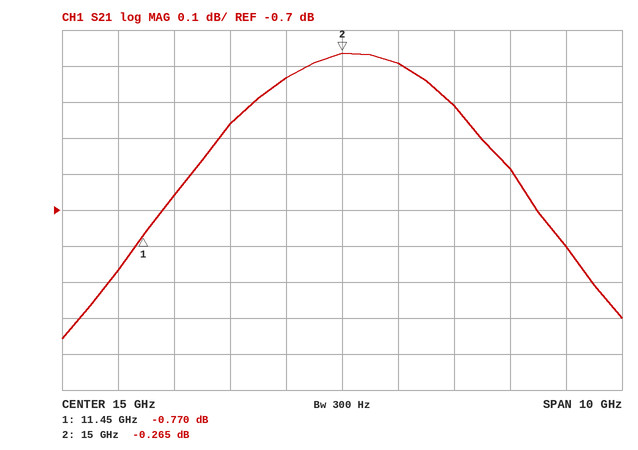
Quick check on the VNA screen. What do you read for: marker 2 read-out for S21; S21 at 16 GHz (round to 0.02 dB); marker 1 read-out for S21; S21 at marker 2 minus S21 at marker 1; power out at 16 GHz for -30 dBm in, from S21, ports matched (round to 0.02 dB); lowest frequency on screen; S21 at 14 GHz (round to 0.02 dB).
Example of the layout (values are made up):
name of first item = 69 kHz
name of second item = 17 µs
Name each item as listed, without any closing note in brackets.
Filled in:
marker 2 read-out for S21 = -0.265 dB
S21 at 16 GHz = -0.30 dB
marker 1 read-out for S21 = -0.770 dB
S21 at marker 2 minus S21 at marker 1 = 0.505 dB
power out at 16 GHz for -30 dBm in, from S21, ports matched = -30.30 dBm
lowest frequency on screen = 10 GHz
S21 at 14 GHz = -0.34 dB
